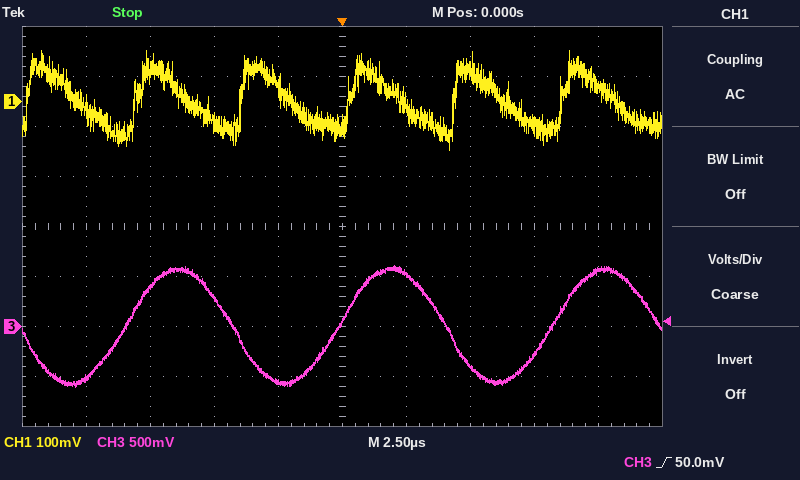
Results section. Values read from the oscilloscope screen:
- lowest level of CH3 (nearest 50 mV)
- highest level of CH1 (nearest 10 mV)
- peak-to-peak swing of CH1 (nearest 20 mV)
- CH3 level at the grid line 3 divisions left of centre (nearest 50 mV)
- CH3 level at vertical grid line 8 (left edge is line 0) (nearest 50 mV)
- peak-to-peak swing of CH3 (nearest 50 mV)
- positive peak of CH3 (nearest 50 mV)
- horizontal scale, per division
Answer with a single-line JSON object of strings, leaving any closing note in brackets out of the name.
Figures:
{"lowest level of CH3": "-600 mV", "highest level of CH1": "100 mV", "peak-to-peak swing of CH1": "200 mV", "CH3 level at the grid line 3 divisions left of centre": "400 mV", "CH3 level at vertical grid line 8 (left edge is line 0)": "-300 mV", "peak-to-peak swing of CH3": "1.20 V", "positive peak of CH3": "600 mV", "horizontal scale, per division": "2.5 µs"}
